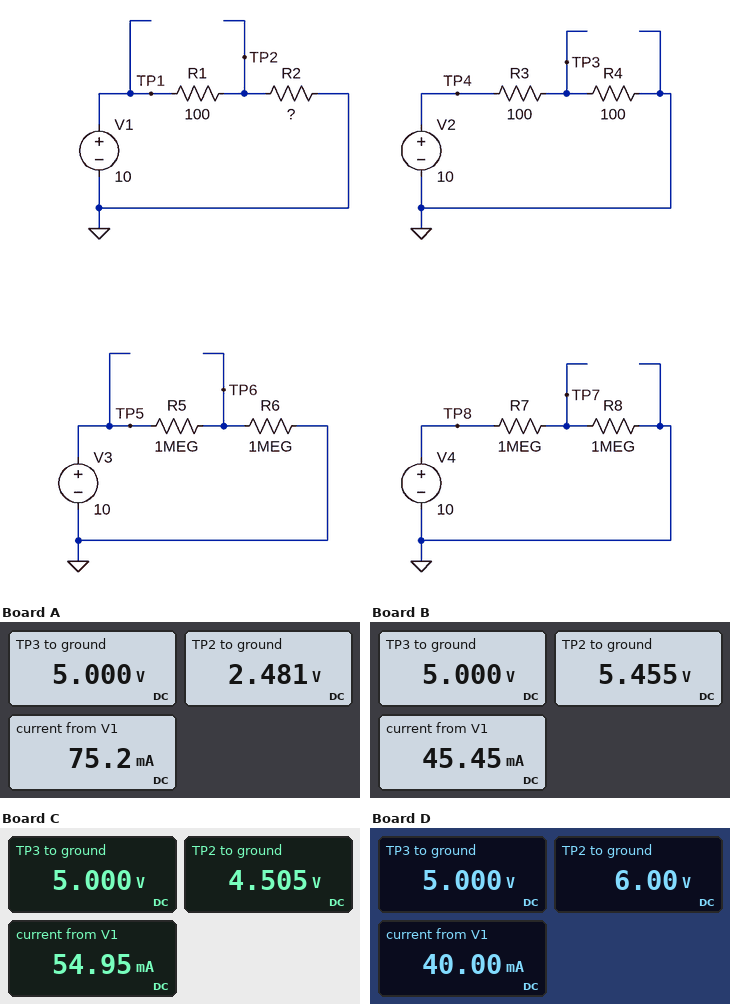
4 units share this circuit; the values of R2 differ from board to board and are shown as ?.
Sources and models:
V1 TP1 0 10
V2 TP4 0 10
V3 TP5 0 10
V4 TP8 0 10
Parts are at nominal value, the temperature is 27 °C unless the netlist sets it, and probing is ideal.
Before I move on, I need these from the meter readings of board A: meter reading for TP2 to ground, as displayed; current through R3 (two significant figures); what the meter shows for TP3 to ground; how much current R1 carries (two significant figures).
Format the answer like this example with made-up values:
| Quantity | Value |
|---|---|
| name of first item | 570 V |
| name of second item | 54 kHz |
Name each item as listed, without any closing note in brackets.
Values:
| Quantity | Value |
|---|---|
| meter reading for TP2 to ground, as displayed | 2.481 V |
| current through R3 | 50 mA |
| what the meter shows for TP3 to ground | 5.000 V |
| how much current R1 carries | 75 mA |
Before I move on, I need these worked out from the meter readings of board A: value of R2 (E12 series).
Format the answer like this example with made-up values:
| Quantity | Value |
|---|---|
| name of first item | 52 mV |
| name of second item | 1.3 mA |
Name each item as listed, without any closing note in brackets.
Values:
| Quantity | Value |
|---|---|
| value of R2 | 33 Ω |
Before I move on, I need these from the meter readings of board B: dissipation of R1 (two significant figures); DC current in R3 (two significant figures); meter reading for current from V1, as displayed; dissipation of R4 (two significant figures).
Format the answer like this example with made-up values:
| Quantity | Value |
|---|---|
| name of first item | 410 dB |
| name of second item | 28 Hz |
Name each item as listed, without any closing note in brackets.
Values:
| Quantity | Value |
|---|---|
| dissipation of R1 | 210 mW |
| DC current in R3 | 50 mA |
| meter reading for current from V1, as displayed | 45.45 mA |
| dissipation of R4 | 250 mW |
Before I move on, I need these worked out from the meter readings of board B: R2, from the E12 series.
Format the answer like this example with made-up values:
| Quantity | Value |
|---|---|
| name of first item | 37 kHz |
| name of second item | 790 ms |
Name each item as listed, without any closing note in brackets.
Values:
| Quantity | Value |
|---|---|
| R2, from the E12 series | 120 Ω |
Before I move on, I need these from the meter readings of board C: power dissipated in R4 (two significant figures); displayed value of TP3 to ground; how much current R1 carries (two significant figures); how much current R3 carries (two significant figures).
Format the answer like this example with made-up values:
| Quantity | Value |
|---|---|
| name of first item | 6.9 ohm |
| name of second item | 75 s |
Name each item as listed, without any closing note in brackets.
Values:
| Quantity | Value |
|---|---|
| power dissipated in R4 | 250 mW |
| displayed value of TP3 to ground | 5.000 V |
| how much current R1 carries | 55 mA |
| how much current R3 carries | 50 mA |
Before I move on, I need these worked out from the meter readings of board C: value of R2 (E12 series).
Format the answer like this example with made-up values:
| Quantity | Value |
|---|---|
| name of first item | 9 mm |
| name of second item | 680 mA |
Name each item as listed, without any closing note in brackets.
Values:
| Quantity | Value |
|---|---|
| value of R2 | 82 Ω |
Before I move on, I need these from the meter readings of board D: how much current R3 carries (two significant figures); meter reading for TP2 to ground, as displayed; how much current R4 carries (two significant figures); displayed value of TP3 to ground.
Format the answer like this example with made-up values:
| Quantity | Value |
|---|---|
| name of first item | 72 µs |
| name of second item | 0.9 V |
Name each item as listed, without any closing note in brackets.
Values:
| Quantity | Value |
|---|---|
| how much current R3 carries | 50 mA |
| meter reading for TP2 to ground, as displayed | 6.00 V |
| how much current R4 carries | 50 mA |
| displayed value of TP3 to ground | 5.000 V |
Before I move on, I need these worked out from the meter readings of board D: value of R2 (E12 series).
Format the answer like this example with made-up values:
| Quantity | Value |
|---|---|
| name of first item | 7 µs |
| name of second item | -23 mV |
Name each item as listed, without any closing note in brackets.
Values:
| Quantity | Value |
|---|---|
| value of R2 | 150 Ω |
